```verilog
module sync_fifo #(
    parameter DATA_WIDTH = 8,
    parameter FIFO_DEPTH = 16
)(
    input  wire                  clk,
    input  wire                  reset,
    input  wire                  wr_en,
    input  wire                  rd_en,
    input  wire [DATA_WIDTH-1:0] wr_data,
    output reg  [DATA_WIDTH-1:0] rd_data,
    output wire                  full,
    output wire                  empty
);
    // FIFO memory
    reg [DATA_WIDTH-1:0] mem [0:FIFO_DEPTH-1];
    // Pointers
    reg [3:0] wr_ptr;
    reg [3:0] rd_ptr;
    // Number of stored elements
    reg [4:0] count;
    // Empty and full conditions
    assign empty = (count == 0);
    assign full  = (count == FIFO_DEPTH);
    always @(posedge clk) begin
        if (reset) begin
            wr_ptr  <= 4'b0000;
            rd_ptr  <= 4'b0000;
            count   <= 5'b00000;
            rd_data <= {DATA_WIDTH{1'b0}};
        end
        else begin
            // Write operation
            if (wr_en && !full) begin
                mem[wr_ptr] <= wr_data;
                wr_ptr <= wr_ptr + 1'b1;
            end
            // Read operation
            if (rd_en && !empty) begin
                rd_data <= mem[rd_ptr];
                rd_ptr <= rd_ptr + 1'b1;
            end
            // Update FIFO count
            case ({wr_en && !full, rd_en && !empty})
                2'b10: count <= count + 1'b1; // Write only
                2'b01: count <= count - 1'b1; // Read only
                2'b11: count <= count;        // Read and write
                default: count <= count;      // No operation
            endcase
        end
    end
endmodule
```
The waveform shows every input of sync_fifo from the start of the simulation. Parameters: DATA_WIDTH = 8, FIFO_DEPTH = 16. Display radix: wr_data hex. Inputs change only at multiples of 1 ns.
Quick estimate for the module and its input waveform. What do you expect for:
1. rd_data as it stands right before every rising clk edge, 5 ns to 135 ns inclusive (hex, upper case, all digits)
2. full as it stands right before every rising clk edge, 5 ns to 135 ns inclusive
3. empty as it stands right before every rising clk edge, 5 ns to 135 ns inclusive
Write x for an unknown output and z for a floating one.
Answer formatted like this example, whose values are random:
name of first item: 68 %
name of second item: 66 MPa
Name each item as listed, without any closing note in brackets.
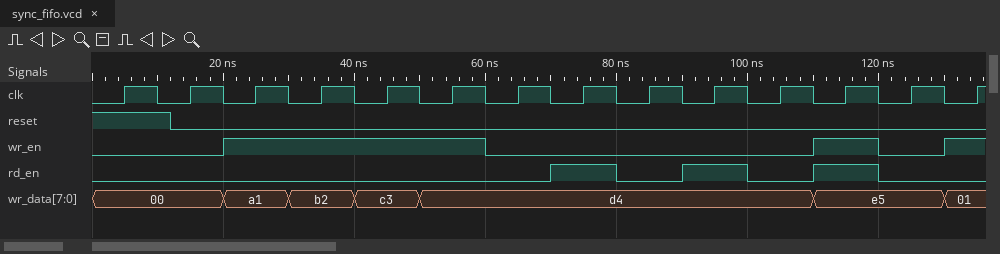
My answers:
rd_data as it stands right before every rising clk edge, 5 ns to 135 ns inclusive: x, 00, 00, 00, 00, 00, 00, 00, A1, A1, B2, B2, C3, C3
full as it stands right before every rising clk edge, 5 ns to 135 ns inclusive: x 0 0 0 0 0 0 0 0 0 0 0 0 0
empty as it stands right before every rising clk edge, 5 ns to 135 ns inclusive: x 1 1 0 0 0 0 0 0 0 0 0 0 0
